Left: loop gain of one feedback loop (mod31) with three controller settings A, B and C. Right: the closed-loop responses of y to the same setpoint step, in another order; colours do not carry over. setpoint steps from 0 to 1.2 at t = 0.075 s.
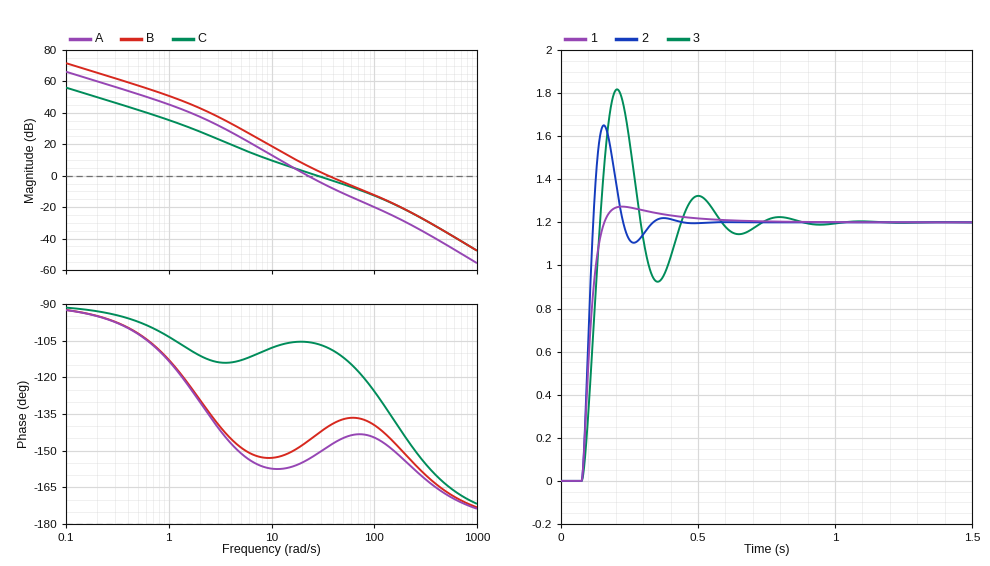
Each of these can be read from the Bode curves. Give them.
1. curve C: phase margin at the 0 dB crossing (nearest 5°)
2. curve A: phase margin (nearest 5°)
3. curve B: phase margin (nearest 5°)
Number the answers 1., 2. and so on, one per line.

1. 75°
2. 25°
3. 40°
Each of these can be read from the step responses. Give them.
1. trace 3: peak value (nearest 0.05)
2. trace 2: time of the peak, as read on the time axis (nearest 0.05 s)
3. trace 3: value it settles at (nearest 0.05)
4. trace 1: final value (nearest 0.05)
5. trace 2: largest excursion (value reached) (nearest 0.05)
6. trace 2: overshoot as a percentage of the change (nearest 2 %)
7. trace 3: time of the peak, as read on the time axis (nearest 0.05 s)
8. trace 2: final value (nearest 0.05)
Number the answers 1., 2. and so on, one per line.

1. 1.80
2. 0.15 s
3. 1.20
4. 1.20
5. 1.65
6. 38 %
7. 0.20 s
8. 1.20
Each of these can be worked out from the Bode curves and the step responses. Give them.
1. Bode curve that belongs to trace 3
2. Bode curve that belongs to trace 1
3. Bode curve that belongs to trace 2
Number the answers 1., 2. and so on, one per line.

1. A
2. C
3. B
